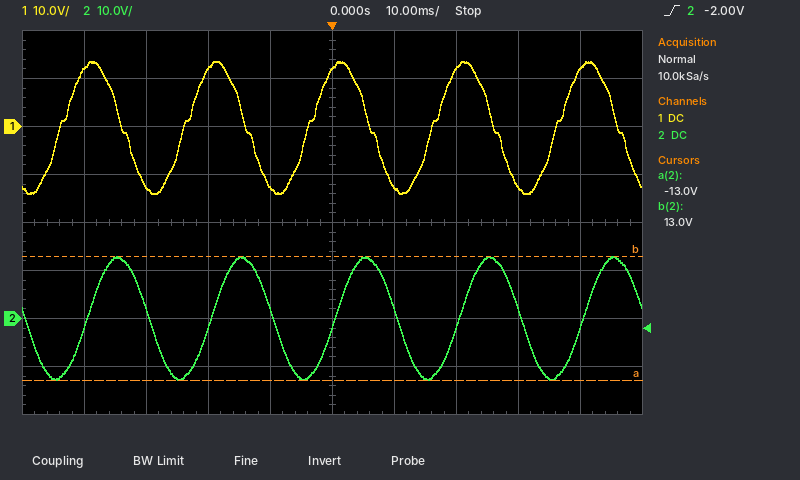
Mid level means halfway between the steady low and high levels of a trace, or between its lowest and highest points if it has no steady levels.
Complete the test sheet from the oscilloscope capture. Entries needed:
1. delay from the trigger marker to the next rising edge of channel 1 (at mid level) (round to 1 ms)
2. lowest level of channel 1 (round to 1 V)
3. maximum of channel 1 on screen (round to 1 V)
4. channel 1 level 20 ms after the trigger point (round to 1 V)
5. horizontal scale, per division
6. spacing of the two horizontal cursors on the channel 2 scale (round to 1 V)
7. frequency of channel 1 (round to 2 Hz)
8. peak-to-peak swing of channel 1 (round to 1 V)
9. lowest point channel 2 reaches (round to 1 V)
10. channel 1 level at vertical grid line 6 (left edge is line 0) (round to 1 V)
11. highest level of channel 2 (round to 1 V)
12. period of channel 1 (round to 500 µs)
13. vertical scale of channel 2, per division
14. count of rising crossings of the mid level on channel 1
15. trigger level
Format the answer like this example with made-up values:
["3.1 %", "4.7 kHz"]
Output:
["16 ms", "-14 V", "14 V", "12 V", "10 ms", "26 V", "50 Hz", "28 V", "-13 V", "-12 V", "13 V", "20.0 ms", "10 V", "5", "-2.00 V"]
